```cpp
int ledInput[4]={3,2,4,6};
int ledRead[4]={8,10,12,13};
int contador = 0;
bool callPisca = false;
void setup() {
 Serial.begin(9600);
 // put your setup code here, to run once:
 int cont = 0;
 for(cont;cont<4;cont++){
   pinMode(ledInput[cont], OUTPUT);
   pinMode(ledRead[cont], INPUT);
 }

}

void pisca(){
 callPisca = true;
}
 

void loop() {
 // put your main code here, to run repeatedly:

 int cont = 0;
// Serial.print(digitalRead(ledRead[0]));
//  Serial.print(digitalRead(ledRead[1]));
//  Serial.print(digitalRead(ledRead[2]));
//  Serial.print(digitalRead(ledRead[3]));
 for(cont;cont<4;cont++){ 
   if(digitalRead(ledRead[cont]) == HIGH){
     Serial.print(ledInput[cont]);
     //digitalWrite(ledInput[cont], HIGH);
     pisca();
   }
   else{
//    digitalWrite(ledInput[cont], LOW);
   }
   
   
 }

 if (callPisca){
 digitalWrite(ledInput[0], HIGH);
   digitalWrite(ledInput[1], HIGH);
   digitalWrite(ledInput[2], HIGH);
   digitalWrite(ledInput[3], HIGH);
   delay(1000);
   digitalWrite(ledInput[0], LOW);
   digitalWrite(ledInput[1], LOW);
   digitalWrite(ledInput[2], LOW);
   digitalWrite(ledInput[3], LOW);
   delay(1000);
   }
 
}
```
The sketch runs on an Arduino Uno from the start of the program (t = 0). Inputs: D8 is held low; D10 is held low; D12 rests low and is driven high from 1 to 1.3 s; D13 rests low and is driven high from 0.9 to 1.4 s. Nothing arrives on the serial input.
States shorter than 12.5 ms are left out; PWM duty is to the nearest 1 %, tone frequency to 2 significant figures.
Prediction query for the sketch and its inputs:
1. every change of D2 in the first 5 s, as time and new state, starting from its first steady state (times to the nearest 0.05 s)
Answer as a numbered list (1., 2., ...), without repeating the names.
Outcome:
1. 0 s low; 0.9 s high; 1.9 s low; 2.9 s high; 3.9 s low; 4.9 s high
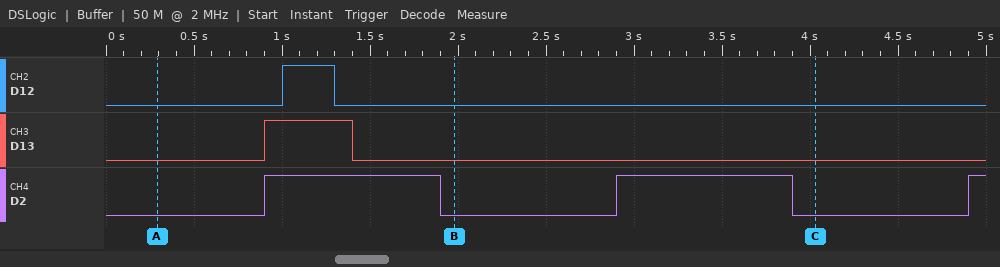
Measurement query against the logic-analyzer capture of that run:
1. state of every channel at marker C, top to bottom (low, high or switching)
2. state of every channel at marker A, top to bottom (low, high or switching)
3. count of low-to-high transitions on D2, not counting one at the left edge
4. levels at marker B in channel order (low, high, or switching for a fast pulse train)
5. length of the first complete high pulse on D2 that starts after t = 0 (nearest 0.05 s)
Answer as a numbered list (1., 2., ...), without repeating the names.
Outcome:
1. D12 low, D13 low, D2 low
2. D12 low, D13 low, D2 low
3. 3
4. D12 low, D13 low, D2 low
5. 1.00 s
